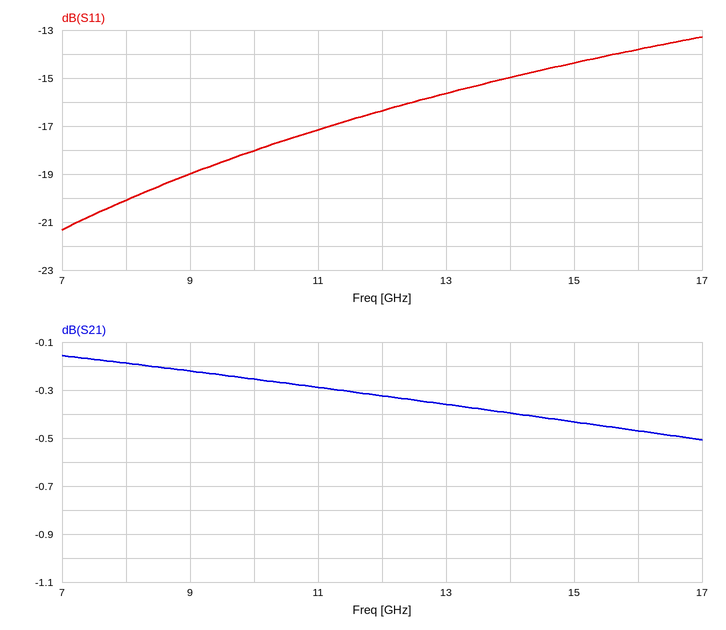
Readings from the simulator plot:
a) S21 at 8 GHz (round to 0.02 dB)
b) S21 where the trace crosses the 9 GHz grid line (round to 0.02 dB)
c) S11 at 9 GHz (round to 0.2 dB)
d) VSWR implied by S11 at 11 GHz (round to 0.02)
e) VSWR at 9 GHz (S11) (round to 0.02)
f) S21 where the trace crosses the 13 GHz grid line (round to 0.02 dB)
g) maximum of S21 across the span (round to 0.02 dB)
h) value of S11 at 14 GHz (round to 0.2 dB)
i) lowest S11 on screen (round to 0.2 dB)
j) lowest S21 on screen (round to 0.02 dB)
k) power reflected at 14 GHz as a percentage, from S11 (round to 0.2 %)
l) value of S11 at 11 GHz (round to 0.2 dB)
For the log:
-0.18 dB
-0.22 dB
-19.0 dB
1.32
1.26
-0.36 dB
-0.16 dB
-15.0 dB
-21.4 dB
-0.50 dB
3.2 %
-17.2 dB
